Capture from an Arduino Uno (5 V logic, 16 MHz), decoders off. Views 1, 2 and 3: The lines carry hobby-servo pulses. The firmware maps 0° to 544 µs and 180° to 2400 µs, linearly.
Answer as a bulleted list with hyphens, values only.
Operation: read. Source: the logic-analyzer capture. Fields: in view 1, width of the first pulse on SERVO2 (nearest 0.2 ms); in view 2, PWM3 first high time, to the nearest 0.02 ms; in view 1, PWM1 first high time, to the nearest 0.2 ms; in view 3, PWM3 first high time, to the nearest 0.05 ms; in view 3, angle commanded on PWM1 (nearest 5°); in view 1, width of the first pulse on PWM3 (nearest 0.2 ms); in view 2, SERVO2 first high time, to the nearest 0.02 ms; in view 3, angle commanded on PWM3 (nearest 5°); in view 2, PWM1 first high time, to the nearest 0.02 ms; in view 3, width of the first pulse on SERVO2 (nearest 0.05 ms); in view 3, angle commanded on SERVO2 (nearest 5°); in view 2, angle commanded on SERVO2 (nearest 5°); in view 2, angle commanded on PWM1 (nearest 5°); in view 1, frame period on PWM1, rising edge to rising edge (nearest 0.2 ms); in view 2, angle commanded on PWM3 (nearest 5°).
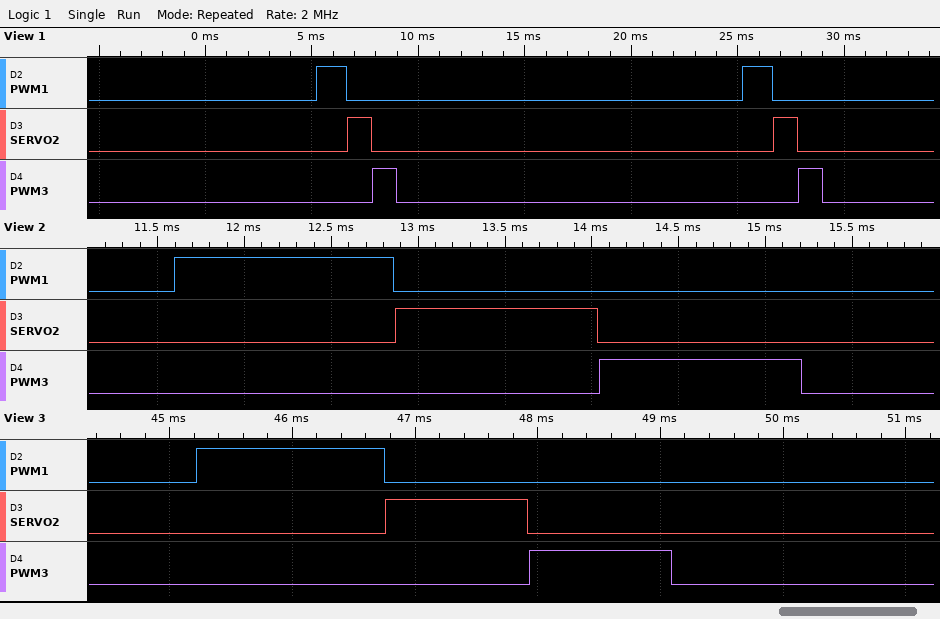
- 1.2 ms
- 1.16 ms
- 1.4 ms
- 1.15 ms
- 95°
- 1.2 ms
- 1.16 ms
- 60°
- 1.26 ms
- 1.15 ms
- 60°
- 60°
- 70°
- 20.0 ms
- 60°
